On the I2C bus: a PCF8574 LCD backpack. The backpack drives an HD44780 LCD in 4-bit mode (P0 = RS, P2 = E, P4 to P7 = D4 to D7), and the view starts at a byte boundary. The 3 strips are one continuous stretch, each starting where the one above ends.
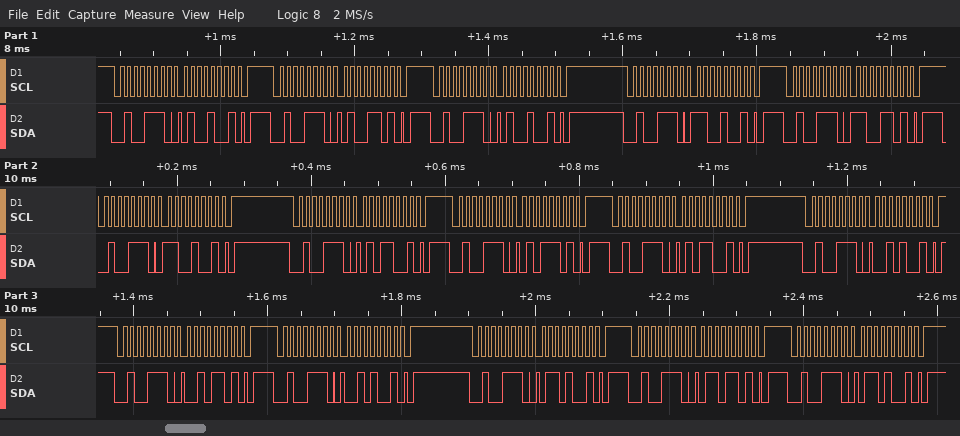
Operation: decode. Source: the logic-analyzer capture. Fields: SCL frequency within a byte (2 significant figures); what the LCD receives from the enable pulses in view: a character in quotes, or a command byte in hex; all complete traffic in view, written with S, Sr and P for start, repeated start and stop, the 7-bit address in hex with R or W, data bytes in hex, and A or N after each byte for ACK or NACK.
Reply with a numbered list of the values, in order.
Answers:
1. 100 kHz
2. 'L' 'R'
3. S 27W A 49 A P S 27W A 4D A P S 27W A 49 A P S 27W A C9 A P S 27W A CD A P S 27W A C9 A P S 27W A 59 A P S 27W A 5D A P S 27W A 59 A P S 27W A 29 A P S 27W A 2D A P S 27W A 29 A P S 27W A 69 A P S 27W A 6D A P S 27W A 69 A P
